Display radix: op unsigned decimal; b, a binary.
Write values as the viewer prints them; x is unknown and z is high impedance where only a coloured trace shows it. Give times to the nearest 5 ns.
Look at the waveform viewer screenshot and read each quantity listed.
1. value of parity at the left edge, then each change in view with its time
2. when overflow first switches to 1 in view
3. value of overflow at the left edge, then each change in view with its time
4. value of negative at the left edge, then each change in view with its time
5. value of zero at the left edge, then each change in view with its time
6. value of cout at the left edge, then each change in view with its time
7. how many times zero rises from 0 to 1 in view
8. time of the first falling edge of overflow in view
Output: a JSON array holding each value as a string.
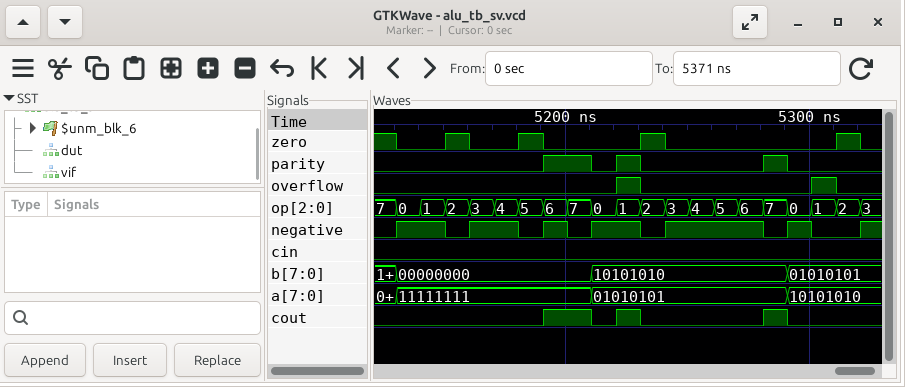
["0, 1 at 5190 ns, 0 at 5210 ns, 1 at 5220 ns, 0 at 5230 ns, 1 at 5280 ns, 0 at 5290 ns", "5220 ns", "0, 1 at 5220 ns, 0 at 5230 ns, 1 at 5300 ns, 0 at 5310 ns", "0, 1 at 5130 ns, 0 at 5150 ns, 1 at 5160 ns, 0 at 5180 ns, 1 at 5190 ns, 0 at 5200 ns, 1 at 5210 ns, 0 at 5230 ns, 1 at 5240 ns, 0 at 5280 ns, 1 at 5290 ns, 0 at 5300 ns, 1 at 5320 ns", "1, 0 at 5130 ns, 1 at 5150 ns, 0 at 5160 ns, 1 at 5180 ns, 0 at 5190 ns, 1 at 5230 ns, 0 at 5240 ns, 1 at 5310 ns, 0 at 5320 ns", "0, 1 at 5190 ns, 0 at 5210 ns, 1 at 5220 ns, 0 at 5230 ns, 1 at 5280 ns, 0 at 5290 ns", "4", "5230 ns"]
